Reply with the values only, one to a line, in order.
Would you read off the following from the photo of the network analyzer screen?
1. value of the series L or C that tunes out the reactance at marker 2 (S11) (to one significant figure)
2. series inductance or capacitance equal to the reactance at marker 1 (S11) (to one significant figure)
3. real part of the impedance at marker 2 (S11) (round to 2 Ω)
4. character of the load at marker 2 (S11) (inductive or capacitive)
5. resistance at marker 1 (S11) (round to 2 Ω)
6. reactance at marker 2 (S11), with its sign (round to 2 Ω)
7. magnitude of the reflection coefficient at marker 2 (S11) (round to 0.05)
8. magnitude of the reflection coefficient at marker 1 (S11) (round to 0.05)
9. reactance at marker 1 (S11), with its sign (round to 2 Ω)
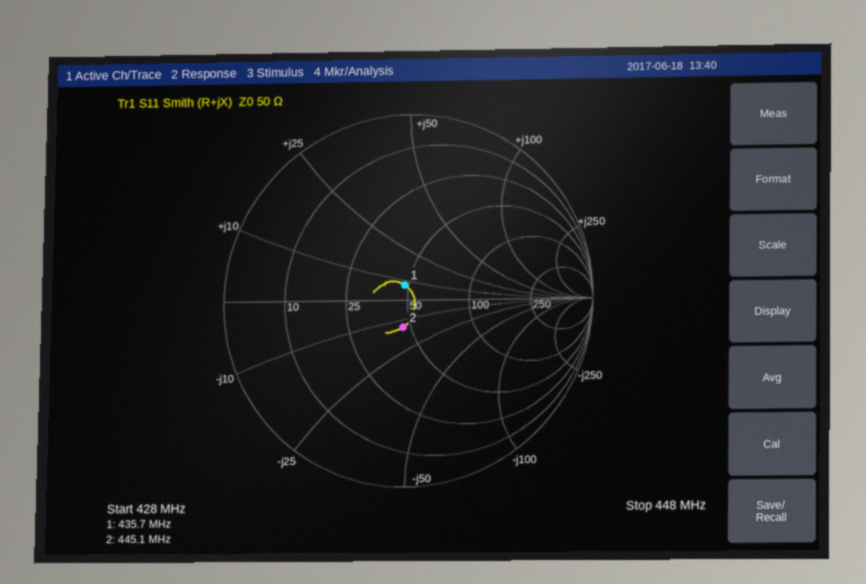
5 nH
3 nH
46 Ω
capacitive
48 Ω
-14 Ω
0.15
0.10
+8 Ω
